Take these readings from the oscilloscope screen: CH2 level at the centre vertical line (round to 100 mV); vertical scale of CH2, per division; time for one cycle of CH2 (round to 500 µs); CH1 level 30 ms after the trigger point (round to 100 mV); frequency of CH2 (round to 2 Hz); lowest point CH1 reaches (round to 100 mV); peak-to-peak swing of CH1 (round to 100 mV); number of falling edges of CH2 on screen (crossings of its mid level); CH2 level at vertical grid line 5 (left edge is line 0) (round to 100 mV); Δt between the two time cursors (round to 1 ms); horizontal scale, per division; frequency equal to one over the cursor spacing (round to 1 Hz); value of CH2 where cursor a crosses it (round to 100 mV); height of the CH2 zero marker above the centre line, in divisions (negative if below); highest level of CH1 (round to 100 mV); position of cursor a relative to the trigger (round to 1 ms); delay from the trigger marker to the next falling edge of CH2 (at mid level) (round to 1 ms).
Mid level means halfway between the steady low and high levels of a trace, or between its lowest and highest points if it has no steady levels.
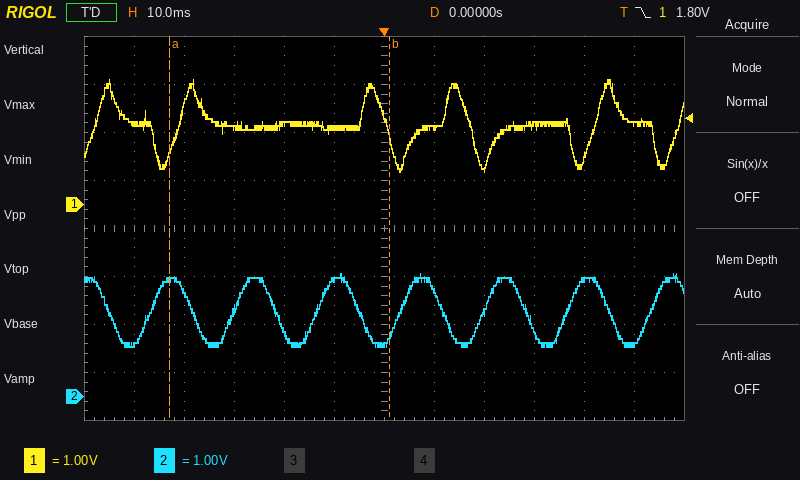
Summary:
1.1 V
1 V
16.5 ms
1.6 V
60 Hz
700 mV
1.9 V
7
2.4 V
44 ms
10 ms
23 Hz
2.4 V
-3.5 div
2.6 V
-43 ms
12 ms
